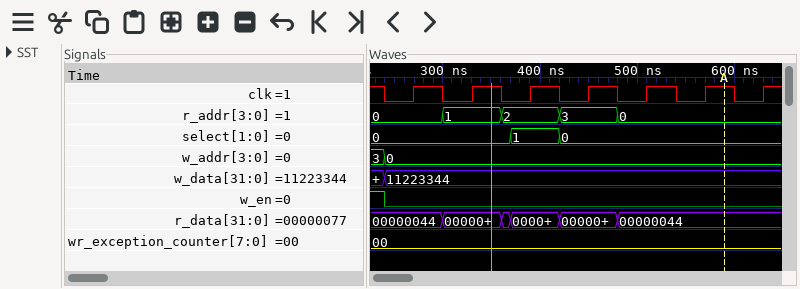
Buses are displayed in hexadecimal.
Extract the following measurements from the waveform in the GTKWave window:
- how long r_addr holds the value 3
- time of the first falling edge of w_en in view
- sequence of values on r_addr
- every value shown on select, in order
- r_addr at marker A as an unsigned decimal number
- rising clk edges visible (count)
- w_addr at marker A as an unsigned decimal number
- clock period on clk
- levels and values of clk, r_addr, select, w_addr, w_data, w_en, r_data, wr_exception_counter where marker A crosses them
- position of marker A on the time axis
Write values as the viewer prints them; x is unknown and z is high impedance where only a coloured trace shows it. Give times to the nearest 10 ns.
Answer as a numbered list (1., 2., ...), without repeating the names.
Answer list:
1. 60 ns
2. 240 ns
3. 0, 1, 2, 3, 0
4. 0, 1, 0
5. 0
6. 7
7. 0
8. 60 ns
9. clk=1, r_addr=0, select=0, w_addr=0, w_data=11223344, w_en=0, r_data=00000044, wr_exception_counter=00
10. 590 ns
